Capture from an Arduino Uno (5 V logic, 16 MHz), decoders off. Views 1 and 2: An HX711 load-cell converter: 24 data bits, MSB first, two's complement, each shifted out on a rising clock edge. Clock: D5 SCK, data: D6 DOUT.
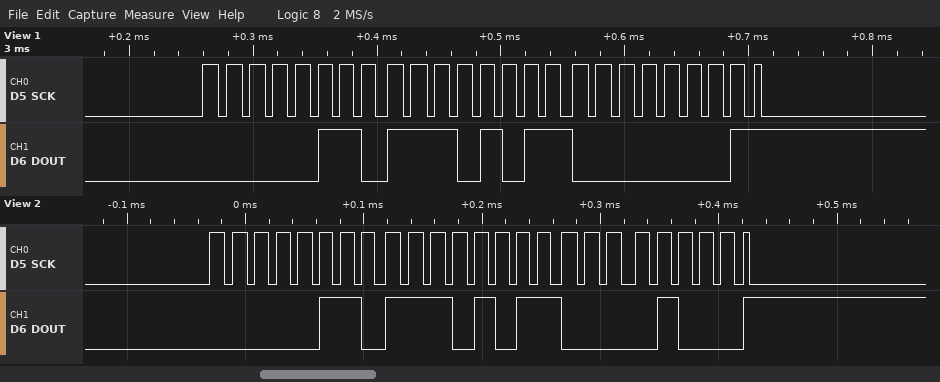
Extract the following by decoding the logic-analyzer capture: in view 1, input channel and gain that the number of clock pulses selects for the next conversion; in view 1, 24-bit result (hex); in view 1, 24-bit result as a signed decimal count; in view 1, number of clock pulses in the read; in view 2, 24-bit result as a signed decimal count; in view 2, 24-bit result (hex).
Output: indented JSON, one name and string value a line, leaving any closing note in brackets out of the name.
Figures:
{
  "in view 1, input channel and gain that the number of clock pulses selects for the next conversion": "channel A, gain 128",
  "in view 1, 24-bit result": "0x06EB01",
  "in view 1, 24-bit result as a signed decimal count": "453377",
  "in view 1, number of clock pulses in the read": "25",
  "in view 2, 24-bit result as a signed decimal count": "453384",
  "in view 2, 24-bit result": "0x06EB08"
}
